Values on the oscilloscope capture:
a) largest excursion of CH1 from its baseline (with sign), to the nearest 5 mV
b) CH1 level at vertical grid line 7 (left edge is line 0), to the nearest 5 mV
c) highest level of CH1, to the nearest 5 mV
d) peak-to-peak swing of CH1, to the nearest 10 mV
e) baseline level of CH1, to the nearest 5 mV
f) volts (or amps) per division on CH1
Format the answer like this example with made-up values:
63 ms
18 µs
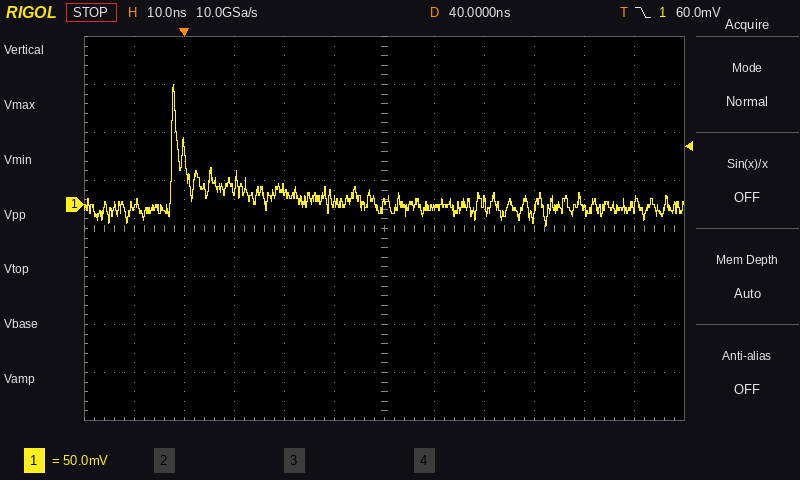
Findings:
+125 mV
-5 mV
125 mV
150 mV
0 mV
50 mV
